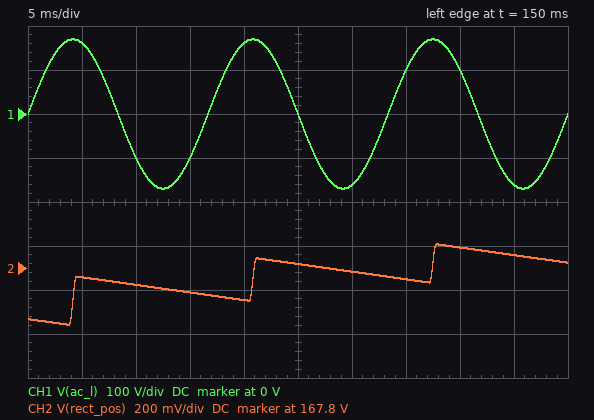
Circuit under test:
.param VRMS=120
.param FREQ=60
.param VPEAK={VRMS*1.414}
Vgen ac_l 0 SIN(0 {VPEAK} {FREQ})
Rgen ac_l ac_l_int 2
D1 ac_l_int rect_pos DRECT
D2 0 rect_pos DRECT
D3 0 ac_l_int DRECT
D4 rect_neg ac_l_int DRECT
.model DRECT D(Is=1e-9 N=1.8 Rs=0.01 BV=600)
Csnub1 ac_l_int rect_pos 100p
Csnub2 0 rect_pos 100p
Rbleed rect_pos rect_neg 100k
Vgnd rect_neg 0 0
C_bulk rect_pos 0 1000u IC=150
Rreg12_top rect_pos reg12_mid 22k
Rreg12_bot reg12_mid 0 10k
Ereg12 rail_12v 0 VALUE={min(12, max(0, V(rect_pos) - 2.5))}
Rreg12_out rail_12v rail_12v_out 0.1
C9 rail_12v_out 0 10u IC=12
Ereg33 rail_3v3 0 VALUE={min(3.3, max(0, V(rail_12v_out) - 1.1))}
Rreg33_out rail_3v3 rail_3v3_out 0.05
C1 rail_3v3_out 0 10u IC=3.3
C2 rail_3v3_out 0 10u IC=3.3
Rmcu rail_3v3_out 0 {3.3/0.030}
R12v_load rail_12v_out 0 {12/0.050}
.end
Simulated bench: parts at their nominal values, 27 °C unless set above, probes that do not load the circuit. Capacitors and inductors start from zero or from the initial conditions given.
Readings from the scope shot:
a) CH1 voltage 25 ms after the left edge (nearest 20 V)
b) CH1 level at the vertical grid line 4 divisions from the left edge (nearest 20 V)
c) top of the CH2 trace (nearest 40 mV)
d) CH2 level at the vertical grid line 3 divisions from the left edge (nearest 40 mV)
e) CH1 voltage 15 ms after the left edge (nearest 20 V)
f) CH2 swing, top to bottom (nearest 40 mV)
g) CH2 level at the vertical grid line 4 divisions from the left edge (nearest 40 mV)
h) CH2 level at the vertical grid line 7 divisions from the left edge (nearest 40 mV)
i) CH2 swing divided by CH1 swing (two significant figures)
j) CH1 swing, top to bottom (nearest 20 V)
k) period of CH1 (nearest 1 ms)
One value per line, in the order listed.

0 V
160 V
167.92 V
167.68 V
-100 V
360 mV
167.64 V
167.76 V
0.0011
340 V
17 ms
